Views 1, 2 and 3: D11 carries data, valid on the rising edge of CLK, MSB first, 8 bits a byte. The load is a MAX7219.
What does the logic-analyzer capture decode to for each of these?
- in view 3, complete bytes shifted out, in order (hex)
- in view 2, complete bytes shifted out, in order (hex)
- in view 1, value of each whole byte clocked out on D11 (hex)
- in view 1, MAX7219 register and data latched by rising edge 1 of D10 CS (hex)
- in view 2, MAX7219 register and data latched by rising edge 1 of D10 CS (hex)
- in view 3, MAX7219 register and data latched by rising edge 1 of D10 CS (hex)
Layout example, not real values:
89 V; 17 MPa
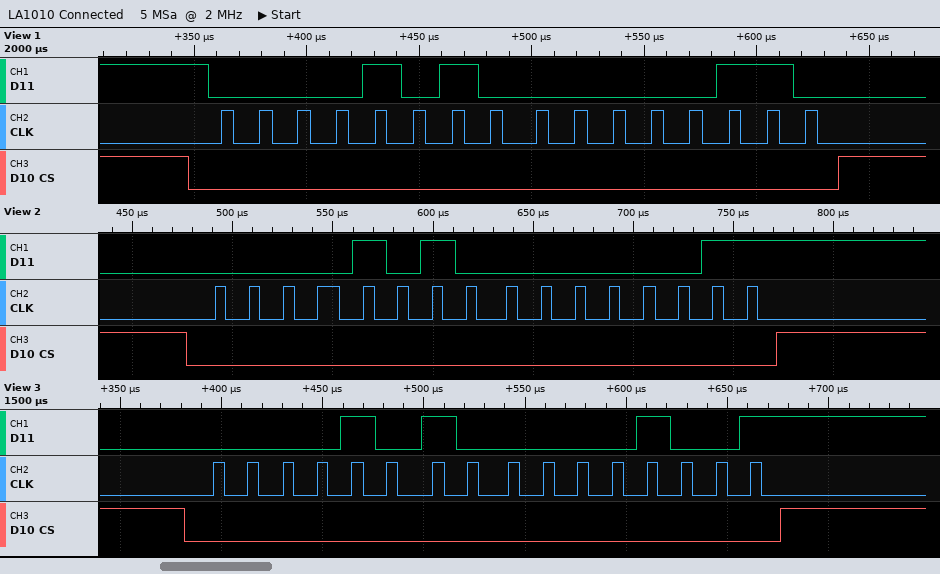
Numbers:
0x0A 0x09; 0A 03; 0A 06; register 0xA, data 0x06; register 0xA, data 0x03; register 0xA, data 0x09
